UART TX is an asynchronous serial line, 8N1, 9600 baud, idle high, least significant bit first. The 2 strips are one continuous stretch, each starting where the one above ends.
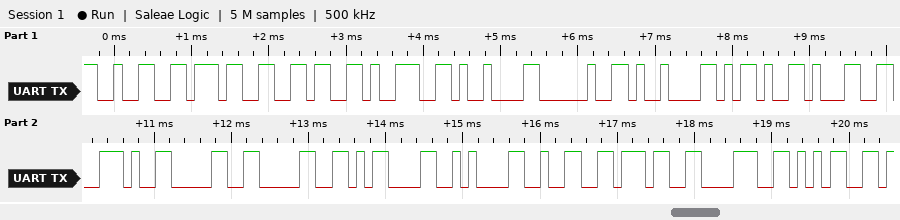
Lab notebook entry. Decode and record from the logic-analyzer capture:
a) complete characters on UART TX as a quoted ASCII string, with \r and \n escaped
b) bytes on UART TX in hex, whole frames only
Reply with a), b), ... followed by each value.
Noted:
a) "2769\t \t-1.00\r\n2785"
b) 0x32 0x37 0x36 0x39 0x09 0x20 0x09 0x2D 0x31 0x2E 0x30 0x30 0x0D 0x0A 0x32 0x37 0x38 0x35
